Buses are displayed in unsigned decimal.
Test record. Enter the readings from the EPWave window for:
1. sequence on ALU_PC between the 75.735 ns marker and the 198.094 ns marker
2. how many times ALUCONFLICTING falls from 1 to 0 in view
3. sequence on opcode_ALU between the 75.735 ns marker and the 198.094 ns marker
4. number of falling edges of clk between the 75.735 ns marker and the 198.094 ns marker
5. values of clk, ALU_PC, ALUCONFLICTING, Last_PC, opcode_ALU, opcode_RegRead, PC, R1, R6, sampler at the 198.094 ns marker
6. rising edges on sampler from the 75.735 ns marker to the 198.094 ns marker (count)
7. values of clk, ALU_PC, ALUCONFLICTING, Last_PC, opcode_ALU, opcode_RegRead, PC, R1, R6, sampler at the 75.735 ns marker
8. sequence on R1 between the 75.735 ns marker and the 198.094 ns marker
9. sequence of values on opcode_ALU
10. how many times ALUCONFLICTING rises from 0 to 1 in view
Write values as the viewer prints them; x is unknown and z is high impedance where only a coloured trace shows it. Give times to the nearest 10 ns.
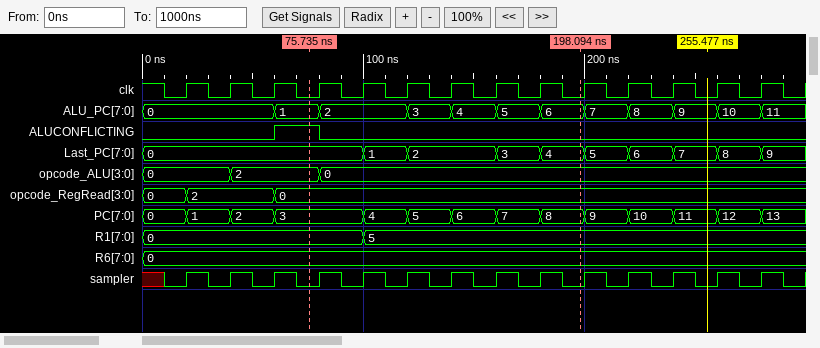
1, 2, 3, 4, 5, 6
1
2, 0
6
clk=0, ALU_PC=6, ALUCONFLICTING=0, Last_PC=4, opcode_ALU=0, opcode_RegRead=0, PC=8, R1=5, R6=0, sampler=0
6
clk=0, ALU_PC=1, ALUCONFLICTING=1, Last_PC=0, opcode_ALU=2, opcode_RegRead=0, PC=3, R1=0, R6=0, sampler=0
0, 5
0, 2, 0
1
